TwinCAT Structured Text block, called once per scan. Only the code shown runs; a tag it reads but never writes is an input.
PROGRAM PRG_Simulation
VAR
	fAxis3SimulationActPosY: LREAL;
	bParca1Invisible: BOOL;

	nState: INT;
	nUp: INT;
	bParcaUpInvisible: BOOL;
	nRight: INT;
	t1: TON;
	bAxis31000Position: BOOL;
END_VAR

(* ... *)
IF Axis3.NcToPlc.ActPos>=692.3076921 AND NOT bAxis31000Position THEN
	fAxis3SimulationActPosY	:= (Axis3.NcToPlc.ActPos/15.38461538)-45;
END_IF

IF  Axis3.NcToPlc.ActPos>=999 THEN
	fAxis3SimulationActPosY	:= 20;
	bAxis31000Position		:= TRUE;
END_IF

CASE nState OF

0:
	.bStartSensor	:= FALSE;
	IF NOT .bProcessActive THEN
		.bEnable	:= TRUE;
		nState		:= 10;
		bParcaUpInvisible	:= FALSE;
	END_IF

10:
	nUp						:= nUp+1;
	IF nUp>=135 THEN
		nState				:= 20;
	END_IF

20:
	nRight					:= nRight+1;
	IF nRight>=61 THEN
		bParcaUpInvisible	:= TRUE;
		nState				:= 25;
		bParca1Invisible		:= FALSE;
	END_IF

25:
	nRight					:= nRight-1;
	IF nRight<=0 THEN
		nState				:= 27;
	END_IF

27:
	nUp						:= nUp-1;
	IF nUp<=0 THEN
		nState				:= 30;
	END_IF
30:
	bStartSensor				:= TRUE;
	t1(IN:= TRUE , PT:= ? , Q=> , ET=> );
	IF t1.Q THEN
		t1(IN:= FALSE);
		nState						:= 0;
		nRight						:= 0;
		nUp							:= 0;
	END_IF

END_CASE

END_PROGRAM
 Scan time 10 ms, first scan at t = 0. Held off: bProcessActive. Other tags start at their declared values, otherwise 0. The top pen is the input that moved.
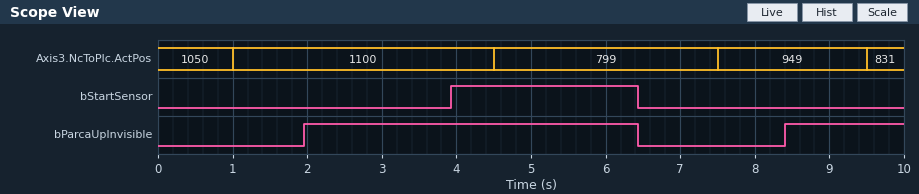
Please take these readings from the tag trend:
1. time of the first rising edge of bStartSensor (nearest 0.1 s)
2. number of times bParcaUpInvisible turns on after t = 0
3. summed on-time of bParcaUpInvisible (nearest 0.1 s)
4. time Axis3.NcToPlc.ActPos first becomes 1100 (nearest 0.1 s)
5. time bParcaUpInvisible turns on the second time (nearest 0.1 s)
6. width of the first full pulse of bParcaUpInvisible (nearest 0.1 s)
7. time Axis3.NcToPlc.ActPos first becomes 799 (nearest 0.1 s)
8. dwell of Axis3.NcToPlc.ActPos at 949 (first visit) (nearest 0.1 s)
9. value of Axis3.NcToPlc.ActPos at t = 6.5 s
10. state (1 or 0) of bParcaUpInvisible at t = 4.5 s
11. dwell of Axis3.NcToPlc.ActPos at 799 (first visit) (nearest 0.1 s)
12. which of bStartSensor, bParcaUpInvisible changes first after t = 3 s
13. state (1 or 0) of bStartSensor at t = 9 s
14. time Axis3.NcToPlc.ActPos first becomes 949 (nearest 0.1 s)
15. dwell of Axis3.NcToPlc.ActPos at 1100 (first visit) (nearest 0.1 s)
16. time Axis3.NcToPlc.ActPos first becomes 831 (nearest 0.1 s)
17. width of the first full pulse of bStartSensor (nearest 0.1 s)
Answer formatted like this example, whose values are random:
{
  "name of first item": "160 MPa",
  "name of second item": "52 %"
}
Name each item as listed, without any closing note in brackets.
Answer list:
{
  "time of the first rising edge of bStartSensor": "3.9 s",
  "number of times bParcaUpInvisible turns on after t = 0": "2",
  "summed on-time of bParcaUpInvisible": "6.1 s",
  "time Axis3.NcToPlc.ActPos first becomes 1100": "1.0 s",
  "time bParcaUpInvisible turns on the second time": "8.4 s",
  "width of the first full pulse of bParcaUpInvisible": "4.5 s",
  "time Axis3.NcToPlc.ActPos first becomes 799": "4.5 s",
  "dwell of Axis3.NcToPlc.ActPos at 949 (first visit)": "2.0 s",
  "value of Axis3.NcToPlc.ActPos at t = 6.5 s": "799",
  "state (1 or 0) of bParcaUpInvisible at t = 4.5 s": "1",
  "dwell of Axis3.NcToPlc.ActPos at 799 (first visit)": "3.0 s",
  "which of bStartSensor, bParcaUpInvisible changes first after t = 3 s": "bStartSensor",
  "state (1 or 0) of bStartSensor at t = 9 s": "0",
  "time Axis3.NcToPlc.ActPos first becomes 949": "7.5 s",
  "dwell of Axis3.NcToPlc.ActPos at 1100 (first visit)": "3.5 s",
  "time Axis3.NcToPlc.ActPos first becomes 831": "9.5 s",
  "width of the first full pulse of bStartSensor": "2.5 s"
}
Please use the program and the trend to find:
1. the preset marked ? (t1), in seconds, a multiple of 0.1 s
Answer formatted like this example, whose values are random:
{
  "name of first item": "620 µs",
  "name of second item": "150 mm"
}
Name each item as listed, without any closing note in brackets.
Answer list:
{
  "the preset marked ? (t1), in seconds, a multiple of 0.1 s": "2.5 s"
}
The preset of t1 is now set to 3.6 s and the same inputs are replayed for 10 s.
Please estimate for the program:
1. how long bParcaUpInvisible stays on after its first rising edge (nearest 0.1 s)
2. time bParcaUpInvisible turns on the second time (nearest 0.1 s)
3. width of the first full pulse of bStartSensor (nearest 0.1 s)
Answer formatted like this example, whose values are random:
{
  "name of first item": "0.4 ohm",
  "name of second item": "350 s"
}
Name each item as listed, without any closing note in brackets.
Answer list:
{
  "how long bParcaUpInvisible stays on after its first rising edge": "5.6 s",
  "time bParcaUpInvisible turns on the second time": "9.5 s",
  "width of the first full pulse of bStartSensor": "3.6 s"
}
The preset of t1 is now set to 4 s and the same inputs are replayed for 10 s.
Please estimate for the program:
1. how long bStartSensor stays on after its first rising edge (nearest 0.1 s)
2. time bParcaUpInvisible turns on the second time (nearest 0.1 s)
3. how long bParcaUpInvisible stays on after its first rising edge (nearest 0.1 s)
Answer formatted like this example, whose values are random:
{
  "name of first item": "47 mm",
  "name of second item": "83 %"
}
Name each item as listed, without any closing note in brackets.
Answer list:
{
  "how long bStartSensor stays on after its first rising edge": "4.0 s",
  "time bParcaUpInvisible turns on the second time": "9.9 s",
  "how long bParcaUpInvisible stays on after its first rising edge": "6.0 s"
}
